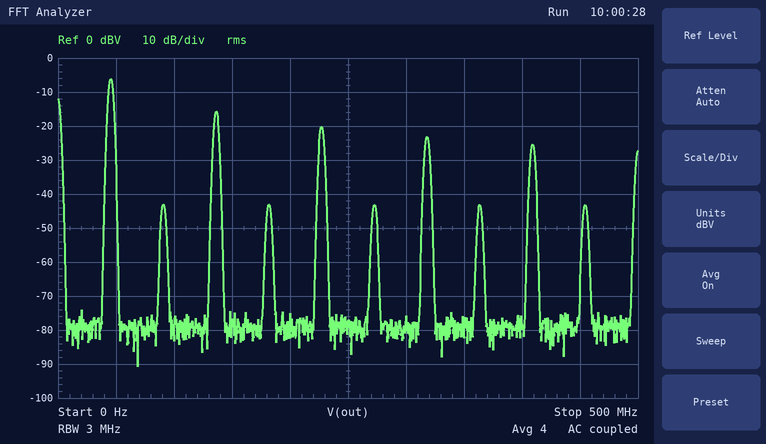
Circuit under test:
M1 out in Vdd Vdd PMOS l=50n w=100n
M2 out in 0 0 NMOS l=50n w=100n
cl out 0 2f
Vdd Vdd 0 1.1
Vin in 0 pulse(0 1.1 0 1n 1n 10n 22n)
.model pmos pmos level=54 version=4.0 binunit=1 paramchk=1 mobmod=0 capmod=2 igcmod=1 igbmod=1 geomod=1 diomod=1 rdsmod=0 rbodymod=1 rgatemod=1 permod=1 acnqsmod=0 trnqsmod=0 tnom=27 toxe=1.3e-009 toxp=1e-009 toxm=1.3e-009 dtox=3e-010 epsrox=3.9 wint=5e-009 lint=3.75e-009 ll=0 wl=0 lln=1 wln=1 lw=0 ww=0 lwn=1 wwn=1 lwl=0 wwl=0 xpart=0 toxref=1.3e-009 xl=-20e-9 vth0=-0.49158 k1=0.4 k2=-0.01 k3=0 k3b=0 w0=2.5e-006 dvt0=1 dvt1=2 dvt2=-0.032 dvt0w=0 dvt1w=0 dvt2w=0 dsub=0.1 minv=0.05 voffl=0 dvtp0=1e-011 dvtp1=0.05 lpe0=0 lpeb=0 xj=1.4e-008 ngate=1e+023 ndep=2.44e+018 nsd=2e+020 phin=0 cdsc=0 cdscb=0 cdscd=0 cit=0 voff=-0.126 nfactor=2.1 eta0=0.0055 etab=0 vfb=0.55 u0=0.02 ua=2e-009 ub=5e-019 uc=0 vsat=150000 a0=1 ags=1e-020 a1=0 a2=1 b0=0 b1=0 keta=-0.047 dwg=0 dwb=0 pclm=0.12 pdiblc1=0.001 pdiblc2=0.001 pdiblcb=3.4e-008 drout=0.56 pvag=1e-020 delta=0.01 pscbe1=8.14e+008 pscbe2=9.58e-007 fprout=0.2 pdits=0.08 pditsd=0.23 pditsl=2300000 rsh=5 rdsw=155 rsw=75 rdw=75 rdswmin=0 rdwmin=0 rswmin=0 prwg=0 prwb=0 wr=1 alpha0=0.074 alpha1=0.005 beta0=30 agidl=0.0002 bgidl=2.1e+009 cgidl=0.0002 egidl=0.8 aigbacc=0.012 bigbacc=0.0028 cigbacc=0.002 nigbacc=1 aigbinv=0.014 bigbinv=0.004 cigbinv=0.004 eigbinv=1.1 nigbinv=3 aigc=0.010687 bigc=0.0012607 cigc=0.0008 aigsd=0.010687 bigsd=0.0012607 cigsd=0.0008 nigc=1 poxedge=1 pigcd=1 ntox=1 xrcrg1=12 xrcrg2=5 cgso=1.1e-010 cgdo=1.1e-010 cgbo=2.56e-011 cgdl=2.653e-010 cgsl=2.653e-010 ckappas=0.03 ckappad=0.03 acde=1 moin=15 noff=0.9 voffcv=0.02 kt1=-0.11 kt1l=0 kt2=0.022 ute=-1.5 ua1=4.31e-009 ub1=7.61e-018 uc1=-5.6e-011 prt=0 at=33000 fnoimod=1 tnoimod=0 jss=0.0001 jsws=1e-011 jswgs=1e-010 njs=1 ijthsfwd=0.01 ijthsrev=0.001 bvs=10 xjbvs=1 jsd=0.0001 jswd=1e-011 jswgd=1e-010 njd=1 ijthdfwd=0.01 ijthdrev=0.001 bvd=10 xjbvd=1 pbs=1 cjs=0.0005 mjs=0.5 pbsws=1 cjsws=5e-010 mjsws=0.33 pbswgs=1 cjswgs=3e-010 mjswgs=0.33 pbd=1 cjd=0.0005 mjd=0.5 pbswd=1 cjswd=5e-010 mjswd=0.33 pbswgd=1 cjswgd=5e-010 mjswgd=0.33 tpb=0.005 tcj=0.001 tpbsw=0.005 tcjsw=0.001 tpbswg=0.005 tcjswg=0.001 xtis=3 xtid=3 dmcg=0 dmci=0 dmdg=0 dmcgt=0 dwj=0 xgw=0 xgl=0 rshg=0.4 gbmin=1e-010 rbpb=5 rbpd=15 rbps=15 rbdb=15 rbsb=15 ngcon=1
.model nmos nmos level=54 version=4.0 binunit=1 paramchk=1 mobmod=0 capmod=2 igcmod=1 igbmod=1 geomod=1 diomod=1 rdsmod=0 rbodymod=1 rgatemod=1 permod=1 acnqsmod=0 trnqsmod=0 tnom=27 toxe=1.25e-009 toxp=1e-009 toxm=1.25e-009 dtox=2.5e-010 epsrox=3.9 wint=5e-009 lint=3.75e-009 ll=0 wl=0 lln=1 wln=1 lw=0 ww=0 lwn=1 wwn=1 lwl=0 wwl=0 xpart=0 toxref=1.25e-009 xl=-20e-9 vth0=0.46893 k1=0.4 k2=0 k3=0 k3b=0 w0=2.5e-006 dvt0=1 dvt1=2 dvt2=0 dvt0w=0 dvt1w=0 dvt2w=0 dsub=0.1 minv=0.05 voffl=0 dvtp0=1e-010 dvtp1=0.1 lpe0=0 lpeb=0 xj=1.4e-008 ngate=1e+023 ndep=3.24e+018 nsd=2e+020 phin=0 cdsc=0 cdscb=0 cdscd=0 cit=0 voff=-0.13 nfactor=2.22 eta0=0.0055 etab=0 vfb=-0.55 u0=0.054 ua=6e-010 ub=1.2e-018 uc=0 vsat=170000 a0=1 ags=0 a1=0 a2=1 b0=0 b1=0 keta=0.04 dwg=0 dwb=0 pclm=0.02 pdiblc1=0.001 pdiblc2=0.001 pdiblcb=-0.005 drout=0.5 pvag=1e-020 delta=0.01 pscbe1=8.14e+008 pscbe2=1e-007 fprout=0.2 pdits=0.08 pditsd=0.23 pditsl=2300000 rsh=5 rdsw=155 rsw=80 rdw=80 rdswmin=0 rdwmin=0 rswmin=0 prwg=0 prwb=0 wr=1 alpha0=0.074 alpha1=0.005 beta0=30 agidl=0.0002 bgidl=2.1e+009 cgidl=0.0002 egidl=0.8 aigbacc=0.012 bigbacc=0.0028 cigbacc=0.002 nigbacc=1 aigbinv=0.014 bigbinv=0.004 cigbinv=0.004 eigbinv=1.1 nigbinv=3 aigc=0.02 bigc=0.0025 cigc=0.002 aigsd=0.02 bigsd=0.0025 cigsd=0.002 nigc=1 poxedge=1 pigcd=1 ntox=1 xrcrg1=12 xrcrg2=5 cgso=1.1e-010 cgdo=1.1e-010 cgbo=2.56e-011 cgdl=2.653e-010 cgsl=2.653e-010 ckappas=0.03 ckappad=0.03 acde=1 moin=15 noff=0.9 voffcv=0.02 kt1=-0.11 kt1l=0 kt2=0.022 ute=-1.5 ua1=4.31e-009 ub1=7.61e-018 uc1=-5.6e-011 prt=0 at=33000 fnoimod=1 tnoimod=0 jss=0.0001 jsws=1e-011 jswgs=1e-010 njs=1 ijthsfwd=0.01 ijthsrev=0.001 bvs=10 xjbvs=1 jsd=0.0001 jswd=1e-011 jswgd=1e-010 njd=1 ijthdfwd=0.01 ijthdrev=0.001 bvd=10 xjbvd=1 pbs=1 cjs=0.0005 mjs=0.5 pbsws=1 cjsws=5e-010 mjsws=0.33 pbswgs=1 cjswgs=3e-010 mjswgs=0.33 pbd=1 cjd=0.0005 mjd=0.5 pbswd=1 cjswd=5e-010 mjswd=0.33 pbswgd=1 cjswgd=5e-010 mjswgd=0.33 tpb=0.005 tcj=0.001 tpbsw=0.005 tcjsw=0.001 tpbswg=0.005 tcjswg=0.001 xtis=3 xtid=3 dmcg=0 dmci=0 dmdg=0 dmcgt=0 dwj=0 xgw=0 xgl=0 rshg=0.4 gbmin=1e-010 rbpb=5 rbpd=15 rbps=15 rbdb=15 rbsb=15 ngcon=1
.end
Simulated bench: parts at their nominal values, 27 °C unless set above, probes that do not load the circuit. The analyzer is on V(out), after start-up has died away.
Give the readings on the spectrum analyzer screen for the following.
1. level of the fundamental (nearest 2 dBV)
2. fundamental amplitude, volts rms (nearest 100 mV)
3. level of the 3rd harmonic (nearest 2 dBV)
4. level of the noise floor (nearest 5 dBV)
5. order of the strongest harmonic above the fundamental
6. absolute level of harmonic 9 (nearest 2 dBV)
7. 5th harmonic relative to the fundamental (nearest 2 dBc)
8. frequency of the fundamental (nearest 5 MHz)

-6 dBV
500 mV
-16 dBV
-80 dBV
3
-26 dBV
-14 dBc
45 MHz
